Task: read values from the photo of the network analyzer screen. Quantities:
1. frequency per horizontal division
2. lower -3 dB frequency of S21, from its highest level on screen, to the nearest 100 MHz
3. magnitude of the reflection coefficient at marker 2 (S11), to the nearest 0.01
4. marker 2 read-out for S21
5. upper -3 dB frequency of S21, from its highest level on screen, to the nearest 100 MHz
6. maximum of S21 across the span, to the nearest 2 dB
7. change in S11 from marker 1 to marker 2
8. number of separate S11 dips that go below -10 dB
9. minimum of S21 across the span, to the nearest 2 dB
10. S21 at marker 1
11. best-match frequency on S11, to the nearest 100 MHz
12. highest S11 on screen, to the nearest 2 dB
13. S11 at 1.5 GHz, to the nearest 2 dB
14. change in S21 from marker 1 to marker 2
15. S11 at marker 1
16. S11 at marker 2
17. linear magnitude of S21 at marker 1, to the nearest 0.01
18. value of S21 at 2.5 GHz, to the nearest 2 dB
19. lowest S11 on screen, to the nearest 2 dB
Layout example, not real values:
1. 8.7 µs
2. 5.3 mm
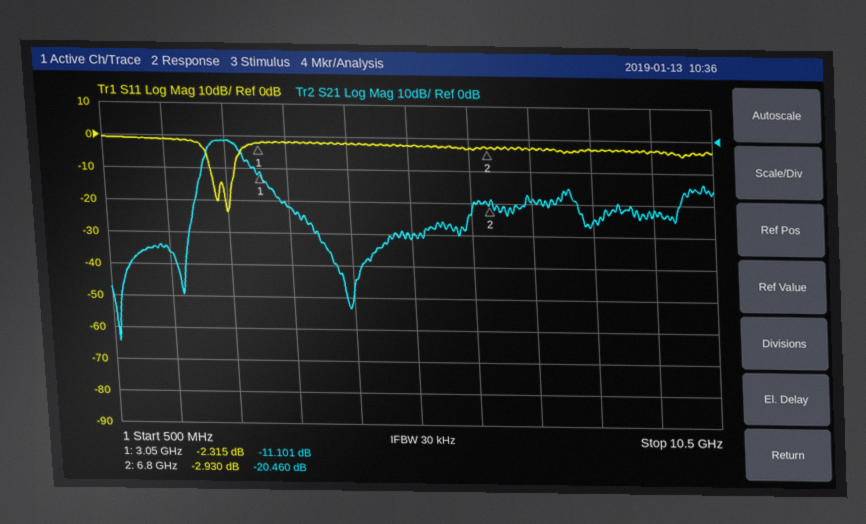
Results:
1. 1 GHz
2. 2.2 GHz
3. 0.71
4. -20.460 dB
5. 2.7 GHz
6. -2 dB
7. -0.615 dB
8. 2
9. -64 dB
10. -11.101 dB
11. 2.5 GHz
12. 0 dB
13. -2 dB
14. -9.359 dB
15. -2.315 dB
16. -2.930 dB
17. 0.28
18. -2 dB
19. -24 dB
